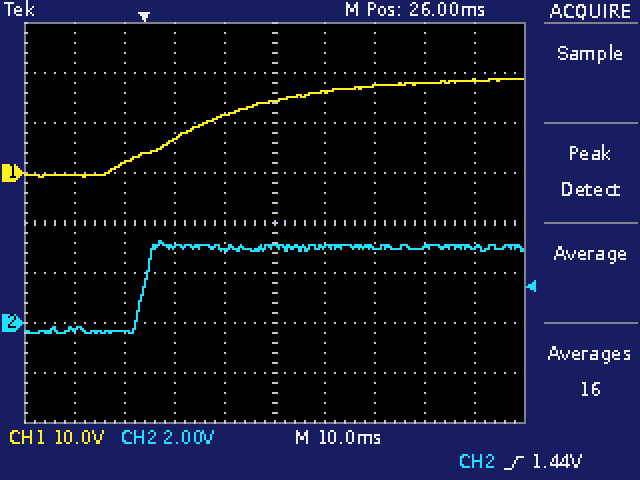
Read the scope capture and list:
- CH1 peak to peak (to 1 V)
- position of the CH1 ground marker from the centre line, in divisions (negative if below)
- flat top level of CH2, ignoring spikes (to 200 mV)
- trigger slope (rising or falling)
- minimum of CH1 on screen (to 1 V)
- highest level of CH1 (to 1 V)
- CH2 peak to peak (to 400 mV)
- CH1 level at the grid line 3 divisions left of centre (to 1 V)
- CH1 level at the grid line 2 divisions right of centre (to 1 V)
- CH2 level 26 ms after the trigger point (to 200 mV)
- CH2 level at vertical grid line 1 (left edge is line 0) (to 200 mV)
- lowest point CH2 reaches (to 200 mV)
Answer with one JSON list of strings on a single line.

["20 V", "+1.0 div", "3.0 V", "rising", "-1 V", "19 V", "3.6 V", "2 V", "17 V", "3.0 V", "-200 mV", "-400 mV"]
